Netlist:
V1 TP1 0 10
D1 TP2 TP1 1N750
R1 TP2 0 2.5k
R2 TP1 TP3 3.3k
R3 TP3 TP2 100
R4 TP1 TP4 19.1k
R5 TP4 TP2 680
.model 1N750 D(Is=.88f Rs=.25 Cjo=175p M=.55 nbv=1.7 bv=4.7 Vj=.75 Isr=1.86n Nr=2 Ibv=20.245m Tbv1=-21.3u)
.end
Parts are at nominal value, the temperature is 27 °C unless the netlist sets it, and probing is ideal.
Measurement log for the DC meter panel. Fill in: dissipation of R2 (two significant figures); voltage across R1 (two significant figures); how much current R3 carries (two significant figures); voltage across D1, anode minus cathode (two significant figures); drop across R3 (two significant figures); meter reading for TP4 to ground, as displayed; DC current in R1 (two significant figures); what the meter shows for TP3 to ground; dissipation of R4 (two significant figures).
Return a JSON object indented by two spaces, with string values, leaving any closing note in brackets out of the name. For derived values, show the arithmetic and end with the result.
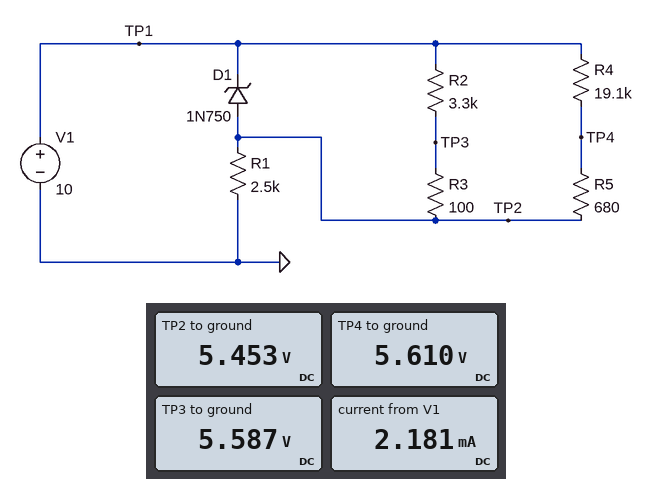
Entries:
{
  "dissipation of R2": "(10 V - 5.587 V)^2 / 3.3 kΩ = 5.9 mW",
  "voltage across R1": "5.453 V = 5.5 V",
  "how much current R3 carries": "(5.587 V - 5.453 V) / 100 Ω = 1.3 mA",
  "voltage across D1, anode minus cathode": "5.453 V - 10 V = -4.5 V",
  "drop across R3": "5.587 V - 5.453 V = 130 mV",
  "meter reading for TP4 to ground, as displayed": "5.610 V",
  "DC current in R1": "(5.453 V) / 2.5 kΩ = 2.2 mA",
  "what the meter shows for TP3 to ground": "5.587 V",
  "dissipation of R4": "(10 V - 5.61 V)^2 / 19.1 kΩ = 1.0 mW"
}
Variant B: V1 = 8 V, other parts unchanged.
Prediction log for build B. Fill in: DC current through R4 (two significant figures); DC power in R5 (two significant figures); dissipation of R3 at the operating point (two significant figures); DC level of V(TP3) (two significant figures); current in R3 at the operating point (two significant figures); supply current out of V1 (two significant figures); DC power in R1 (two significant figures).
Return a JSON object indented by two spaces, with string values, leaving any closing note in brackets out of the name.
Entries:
{
  "DC current through R4": "220 µA",
  "DC power in R5": "32 µW",
  "dissipation of R3 at the operating point": "160 µW",
  "DC level of V(TP3)": "3.8 V",
  "current in R3 at the operating point": "1.3 mA",
  "supply current out of V1": "1.5 mA",
  "DC power in R1": "5.5 mW"
}
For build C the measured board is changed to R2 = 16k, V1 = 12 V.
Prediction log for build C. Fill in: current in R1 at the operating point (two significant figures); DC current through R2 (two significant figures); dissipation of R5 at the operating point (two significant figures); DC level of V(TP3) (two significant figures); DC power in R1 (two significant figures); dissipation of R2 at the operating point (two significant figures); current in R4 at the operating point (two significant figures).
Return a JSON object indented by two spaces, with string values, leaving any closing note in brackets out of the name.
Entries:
{
  "current in R1 at the operating point": "3.0 mA",
  "DC current through R2": "290 µA",
  "dissipation of R5 at the operating point": "37 µW",
  "DC level of V(TP3)": "7.4 V",
  "DC power in R1": "22 mW",
  "dissipation of R2 at the operating point": "1.3 mW",
  "current in R4 at the operating point": "230 µA"
}
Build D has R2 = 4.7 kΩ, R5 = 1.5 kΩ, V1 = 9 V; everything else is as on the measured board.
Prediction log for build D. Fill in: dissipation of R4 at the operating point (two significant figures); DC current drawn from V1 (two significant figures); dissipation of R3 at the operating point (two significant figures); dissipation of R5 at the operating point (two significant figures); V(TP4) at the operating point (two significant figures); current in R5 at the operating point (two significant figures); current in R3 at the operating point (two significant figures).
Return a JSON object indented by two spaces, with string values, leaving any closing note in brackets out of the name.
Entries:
{
  "dissipation of R4 at the operating point": "930 µW",
  "DC current drawn from V1": "1.8 mA",
  "dissipation of R3 at the operating point": "90 µW",
  "dissipation of R5 at the operating point": "73 µW",
  "V(TP4) at the operating point": "4.8 V",
  "current in R5 at the operating point": "220 µA",
  "current in R3 at the operating point": "950 µA"
}
